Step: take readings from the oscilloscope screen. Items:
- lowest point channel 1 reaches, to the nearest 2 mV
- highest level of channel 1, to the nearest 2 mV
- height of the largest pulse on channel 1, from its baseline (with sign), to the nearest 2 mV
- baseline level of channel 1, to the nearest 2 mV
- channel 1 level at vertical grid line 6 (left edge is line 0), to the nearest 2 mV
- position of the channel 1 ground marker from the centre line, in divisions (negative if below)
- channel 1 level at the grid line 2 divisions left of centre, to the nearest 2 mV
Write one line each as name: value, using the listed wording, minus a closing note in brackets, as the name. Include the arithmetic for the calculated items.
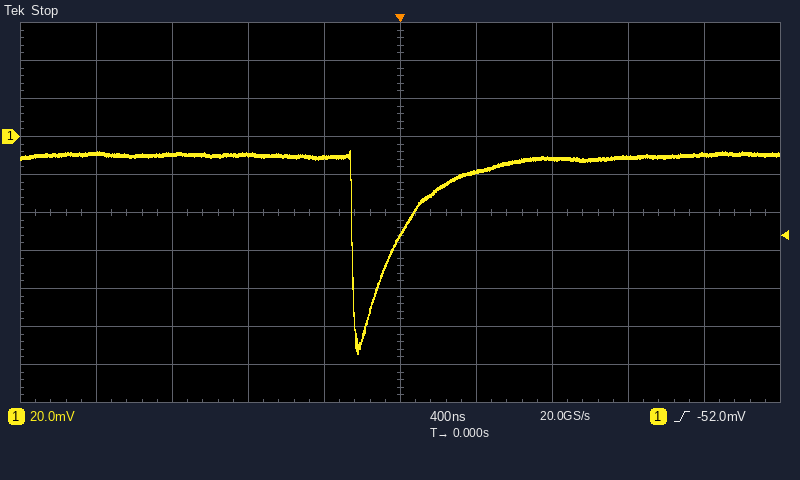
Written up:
lowest point channel 1 reaches, to the nearest 2 mV: -114 mV
highest level of channel 1, to the nearest 2 mV: -8 mV
height of the largest pulse on channel 1, from its baseline (with sign), to the nearest 2 mV: -114 mV − (-10 mV) = -104 mV
baseline level of channel 1, to the nearest 2 mV: -10 mV
channel 1 level at vertical grid line 6 (left edge is line 0), to the nearest 2 mV: -18 mV
position of the channel 1 ground marker from the centre line, in divisions: +2.0 div
channel 1 level at the grid line 2 divisions left of centre, to the nearest 2 mV: -10 mV
